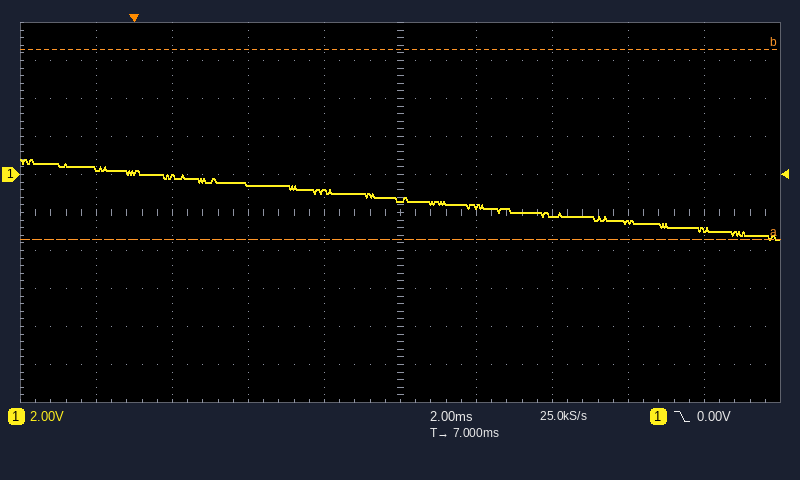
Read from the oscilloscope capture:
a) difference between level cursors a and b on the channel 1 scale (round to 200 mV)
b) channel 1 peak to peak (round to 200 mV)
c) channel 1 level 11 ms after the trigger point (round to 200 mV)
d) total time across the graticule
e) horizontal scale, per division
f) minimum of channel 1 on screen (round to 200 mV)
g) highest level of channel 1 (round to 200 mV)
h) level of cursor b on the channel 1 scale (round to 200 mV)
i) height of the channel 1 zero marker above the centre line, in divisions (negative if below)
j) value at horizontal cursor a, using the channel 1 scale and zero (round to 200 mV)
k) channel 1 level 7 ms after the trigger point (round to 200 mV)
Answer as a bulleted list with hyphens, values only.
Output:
- 10.0 V
- 4.2 V
- -2.2 V
- 20 ms
- 2 ms
- -3.4 V
- 800 mV
- 6.6 V
- +1.0 div
- -3.4 V
- -1.4 V
